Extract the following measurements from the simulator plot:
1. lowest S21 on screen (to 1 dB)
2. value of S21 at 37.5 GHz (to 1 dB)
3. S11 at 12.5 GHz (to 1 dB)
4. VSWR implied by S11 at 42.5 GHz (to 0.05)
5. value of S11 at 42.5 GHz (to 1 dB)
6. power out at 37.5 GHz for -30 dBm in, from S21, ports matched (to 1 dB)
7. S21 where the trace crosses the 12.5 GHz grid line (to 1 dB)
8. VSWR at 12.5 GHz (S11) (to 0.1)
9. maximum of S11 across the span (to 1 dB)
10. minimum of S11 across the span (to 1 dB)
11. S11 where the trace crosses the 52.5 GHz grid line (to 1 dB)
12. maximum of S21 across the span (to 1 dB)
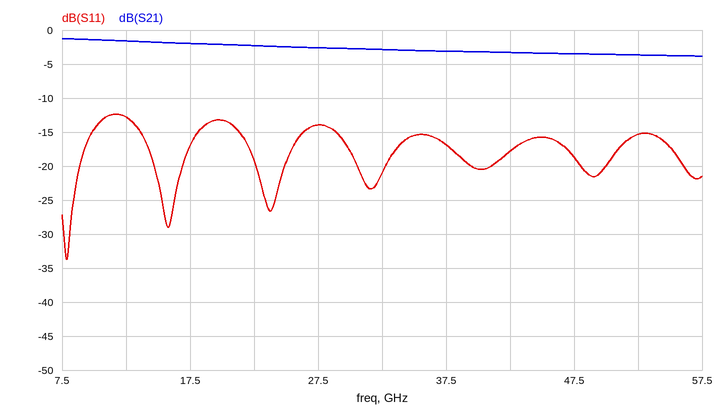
-4 dB
-3 dB
-13 dB
1.30
-18 dB
-33 dBm
-2 dB
1.6
-12 dB
-34 dB
-15 dB
-1 dB
